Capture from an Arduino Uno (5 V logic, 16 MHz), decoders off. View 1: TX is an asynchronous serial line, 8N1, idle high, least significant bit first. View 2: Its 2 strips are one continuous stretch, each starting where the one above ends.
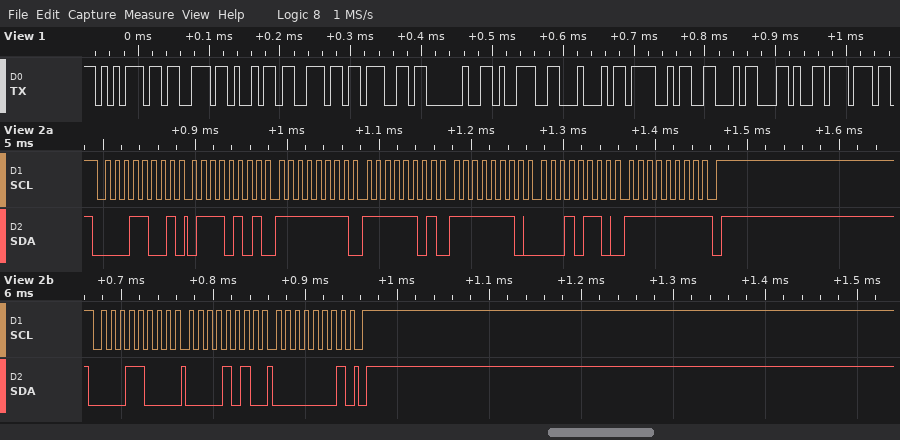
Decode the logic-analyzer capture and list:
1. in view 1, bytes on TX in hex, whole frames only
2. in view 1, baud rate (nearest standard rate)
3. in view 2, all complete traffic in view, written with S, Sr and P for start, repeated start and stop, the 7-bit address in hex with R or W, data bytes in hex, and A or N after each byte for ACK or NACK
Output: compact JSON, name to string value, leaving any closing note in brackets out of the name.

{"in view 1, bytes on TX in hex, whole frames only": "75 73 69 6E 67 20 39 44 4F 46 2C 77", "in view 1, baud rate": "115200 baud", "in view 2, all complete traffic in view, written with S, Sr and P for start, repeated start and stop, the 7-bit address in hex with R or W, data bytes in hex, and A or N after each byte for ACK or NACK": "S 0CR A 75 A FF A FD A FE A 16 A FF N P S 0CW A 0A A 01 A P"}
